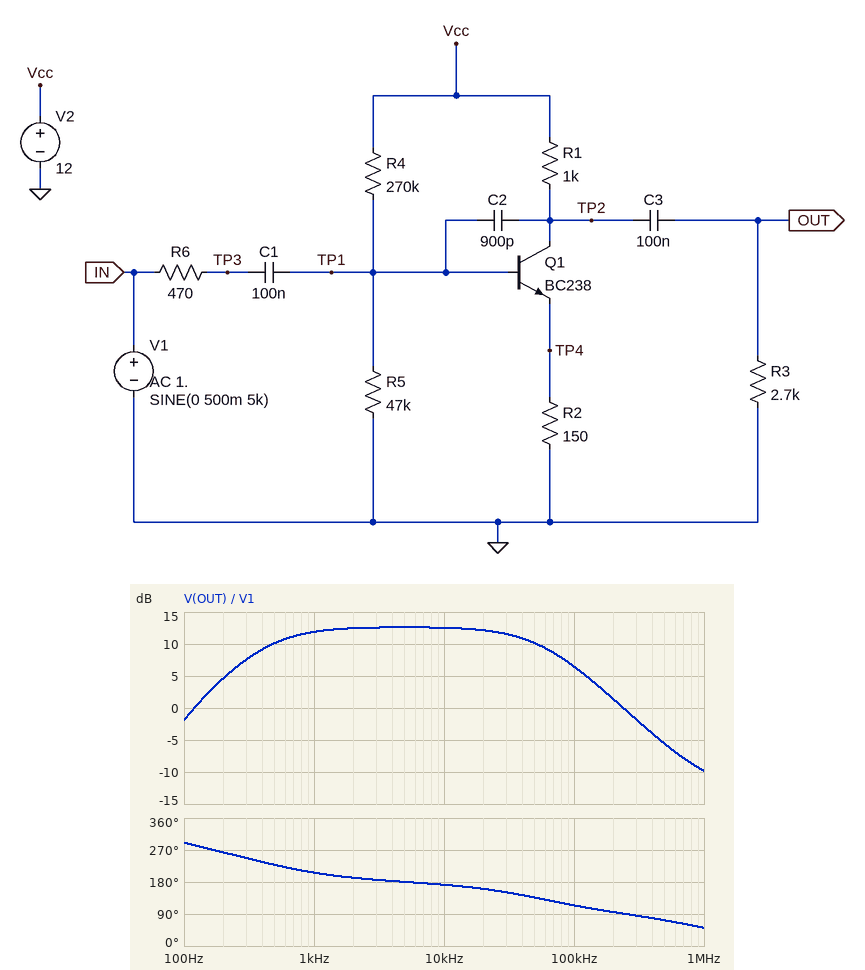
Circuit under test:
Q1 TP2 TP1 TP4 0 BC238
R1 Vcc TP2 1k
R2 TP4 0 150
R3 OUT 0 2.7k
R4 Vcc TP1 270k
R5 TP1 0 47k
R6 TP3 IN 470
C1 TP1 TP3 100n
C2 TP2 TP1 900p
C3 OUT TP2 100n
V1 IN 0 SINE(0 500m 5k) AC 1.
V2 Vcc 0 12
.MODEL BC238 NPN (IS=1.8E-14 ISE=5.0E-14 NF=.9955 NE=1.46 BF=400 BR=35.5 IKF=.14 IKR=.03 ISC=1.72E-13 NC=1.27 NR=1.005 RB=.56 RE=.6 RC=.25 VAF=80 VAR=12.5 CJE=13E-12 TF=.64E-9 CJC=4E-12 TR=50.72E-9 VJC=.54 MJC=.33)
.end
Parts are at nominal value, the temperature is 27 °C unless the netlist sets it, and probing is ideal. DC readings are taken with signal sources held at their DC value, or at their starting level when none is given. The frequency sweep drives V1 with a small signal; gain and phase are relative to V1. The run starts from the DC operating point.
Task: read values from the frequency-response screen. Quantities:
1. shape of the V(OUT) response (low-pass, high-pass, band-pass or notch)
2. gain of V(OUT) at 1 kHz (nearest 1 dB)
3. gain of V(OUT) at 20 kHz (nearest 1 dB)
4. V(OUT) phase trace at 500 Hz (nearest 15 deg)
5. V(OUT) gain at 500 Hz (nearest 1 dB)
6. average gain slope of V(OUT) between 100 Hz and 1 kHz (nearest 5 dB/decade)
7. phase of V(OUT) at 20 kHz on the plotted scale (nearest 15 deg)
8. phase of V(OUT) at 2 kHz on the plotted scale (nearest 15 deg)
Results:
band-pass
12 dB
12 dB
225 deg
10 dB
15 dB/decade
165 deg
195 deg
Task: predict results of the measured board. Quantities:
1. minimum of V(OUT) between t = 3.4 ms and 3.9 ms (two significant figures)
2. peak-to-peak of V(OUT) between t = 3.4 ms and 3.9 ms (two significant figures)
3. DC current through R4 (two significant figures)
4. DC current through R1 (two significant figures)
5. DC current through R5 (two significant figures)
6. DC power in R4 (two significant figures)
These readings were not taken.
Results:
-2.1 V
4.2 V
40 µA
4.0 mA
27 µA
430 µW
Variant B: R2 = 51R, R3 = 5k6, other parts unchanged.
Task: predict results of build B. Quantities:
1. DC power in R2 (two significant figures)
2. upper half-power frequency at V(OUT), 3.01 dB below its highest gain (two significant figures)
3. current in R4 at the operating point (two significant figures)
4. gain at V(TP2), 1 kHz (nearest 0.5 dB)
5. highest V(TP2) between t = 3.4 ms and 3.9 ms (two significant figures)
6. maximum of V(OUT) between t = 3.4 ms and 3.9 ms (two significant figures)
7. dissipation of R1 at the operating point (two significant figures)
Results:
1.9 mW
25 kHz
41 µA
22.0 dB
11 V
4.8 V
37 mW
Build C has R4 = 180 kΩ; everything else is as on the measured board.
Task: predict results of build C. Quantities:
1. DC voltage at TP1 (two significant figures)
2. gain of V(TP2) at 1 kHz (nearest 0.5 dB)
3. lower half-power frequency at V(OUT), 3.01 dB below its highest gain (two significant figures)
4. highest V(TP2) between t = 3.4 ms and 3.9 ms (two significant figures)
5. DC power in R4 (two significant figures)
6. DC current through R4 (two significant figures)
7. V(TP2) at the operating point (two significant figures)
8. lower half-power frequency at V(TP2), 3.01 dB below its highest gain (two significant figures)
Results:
1.7 V
13.5 dB
440 Hz
7.6 V
590 µW
57 µA
5.4 V
61 Hz
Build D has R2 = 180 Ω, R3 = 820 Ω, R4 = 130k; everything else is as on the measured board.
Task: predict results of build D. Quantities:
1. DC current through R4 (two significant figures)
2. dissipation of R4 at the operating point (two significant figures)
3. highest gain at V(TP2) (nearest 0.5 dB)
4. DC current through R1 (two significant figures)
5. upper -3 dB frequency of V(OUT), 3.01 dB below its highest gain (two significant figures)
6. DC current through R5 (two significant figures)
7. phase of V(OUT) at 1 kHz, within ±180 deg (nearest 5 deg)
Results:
75 µA
740 µW
13.5 dB
8.4 mA
93 kHz
47 µA
-135 deg
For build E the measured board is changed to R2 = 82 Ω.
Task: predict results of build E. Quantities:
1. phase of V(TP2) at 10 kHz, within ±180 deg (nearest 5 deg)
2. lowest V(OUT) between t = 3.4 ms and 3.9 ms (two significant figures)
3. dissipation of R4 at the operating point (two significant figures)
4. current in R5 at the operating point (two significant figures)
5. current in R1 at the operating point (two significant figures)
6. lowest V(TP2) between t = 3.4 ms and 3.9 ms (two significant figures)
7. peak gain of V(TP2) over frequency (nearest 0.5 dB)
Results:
165 deg
-3.6 V
440 µW
24 µA
5.2 mA
3.1 V
19.0 dB
